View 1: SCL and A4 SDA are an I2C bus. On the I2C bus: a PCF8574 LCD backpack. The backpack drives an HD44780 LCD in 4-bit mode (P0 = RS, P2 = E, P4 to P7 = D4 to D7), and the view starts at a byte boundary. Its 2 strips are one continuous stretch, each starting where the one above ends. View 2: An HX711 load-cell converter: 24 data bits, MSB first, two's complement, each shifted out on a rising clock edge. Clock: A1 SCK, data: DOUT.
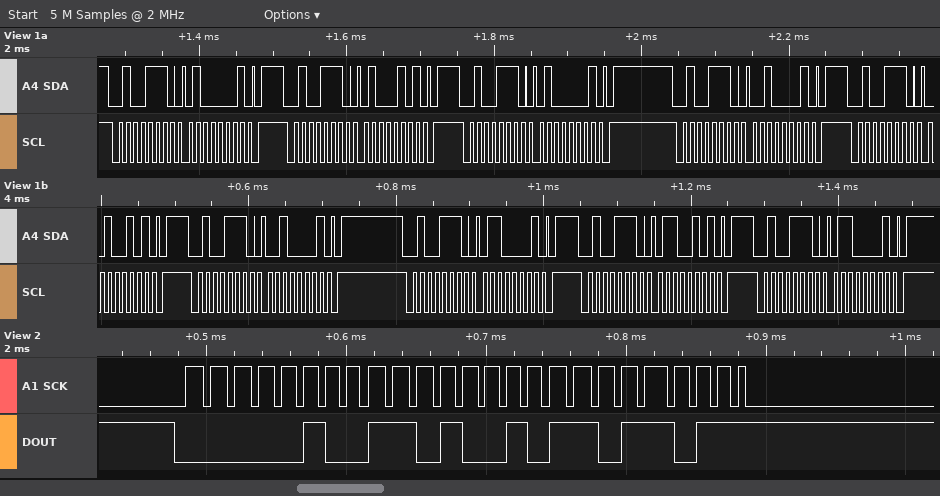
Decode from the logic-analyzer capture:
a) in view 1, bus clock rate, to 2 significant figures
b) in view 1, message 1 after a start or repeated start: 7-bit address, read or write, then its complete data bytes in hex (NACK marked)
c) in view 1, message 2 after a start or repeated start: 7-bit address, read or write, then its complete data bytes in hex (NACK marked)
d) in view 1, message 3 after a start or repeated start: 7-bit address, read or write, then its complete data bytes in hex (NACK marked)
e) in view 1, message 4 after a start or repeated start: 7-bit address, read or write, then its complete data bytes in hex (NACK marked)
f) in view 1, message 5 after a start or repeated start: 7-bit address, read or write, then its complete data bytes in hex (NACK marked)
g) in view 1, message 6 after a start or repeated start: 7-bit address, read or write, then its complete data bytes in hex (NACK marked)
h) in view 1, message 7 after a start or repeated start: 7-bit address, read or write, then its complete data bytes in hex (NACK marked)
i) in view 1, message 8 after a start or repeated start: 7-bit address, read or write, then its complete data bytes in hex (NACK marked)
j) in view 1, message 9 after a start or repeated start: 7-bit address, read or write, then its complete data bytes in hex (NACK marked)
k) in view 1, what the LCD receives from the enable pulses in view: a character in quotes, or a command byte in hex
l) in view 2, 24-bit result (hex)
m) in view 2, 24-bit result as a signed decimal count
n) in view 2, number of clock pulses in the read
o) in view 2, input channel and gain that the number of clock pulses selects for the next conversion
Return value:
100 kHz
0x27 write: 41
0x27 write: 45
0x27 write: 41
0x27 write: 21
0x27 write: 25
0x27 write: 21
0x27 write: 61
0x27 write: 65
0x27 write: 61
'B'
0x04D2DB
316123
25
channel A, gain 128
